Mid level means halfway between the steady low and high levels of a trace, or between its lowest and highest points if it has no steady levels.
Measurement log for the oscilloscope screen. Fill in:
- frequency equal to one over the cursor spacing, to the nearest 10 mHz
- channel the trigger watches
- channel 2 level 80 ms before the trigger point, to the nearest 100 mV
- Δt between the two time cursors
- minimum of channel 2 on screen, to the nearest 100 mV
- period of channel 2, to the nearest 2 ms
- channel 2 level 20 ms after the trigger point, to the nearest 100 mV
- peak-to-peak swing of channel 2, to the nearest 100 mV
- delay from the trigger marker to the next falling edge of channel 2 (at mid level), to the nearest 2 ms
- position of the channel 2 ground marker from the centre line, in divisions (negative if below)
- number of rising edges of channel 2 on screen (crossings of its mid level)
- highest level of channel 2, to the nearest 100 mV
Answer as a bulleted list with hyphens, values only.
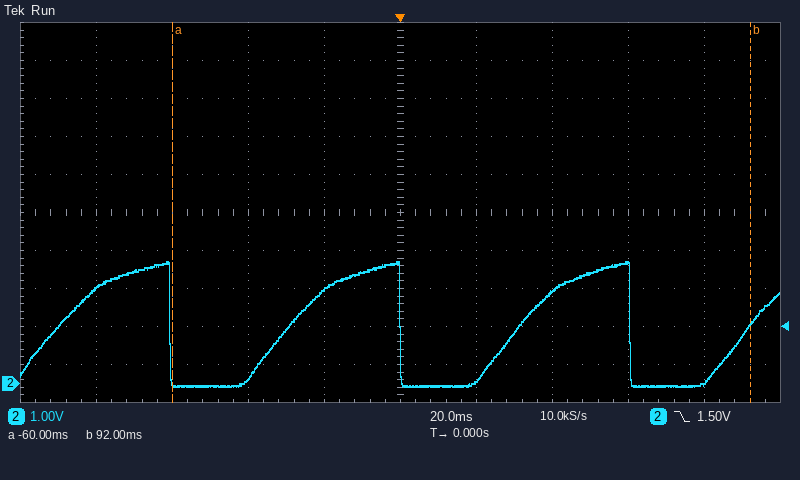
- 6.58 Hz
- channel 2
- 2.5 V
- 152 ms
- -100 mV
- 60 ms
- 100 mV
- 3.3 V
- 60 ms
- -4.5 div
- 4
- 3.2 V
